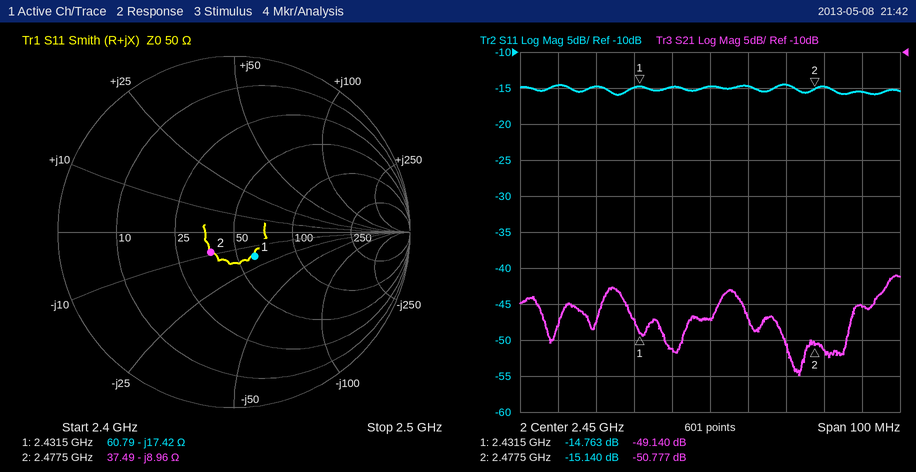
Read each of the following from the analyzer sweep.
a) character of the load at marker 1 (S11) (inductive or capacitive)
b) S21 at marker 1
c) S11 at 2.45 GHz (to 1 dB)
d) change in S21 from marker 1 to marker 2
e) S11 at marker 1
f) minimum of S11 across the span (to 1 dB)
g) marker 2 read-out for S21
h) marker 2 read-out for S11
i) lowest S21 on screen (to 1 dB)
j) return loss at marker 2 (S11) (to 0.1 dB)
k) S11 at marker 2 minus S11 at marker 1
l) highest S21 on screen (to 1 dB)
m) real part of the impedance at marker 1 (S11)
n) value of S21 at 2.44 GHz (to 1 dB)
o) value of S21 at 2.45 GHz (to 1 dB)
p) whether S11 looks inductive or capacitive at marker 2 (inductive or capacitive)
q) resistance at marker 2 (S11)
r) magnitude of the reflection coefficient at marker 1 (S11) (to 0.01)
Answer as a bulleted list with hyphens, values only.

- capacitive
- -49.140 dB
- -15 dB
- -1.637 dB
- -14.763 dB
- -16 dB
- -50.777 dB
- -15.140 dB
- -55 dB
- 15.1 dB
- -0.377 dB
- -41 dB
- 60.79 Ω
- -51 dB
- -47 dB
- capacitive
- 37.49 Ω
- 0.18
